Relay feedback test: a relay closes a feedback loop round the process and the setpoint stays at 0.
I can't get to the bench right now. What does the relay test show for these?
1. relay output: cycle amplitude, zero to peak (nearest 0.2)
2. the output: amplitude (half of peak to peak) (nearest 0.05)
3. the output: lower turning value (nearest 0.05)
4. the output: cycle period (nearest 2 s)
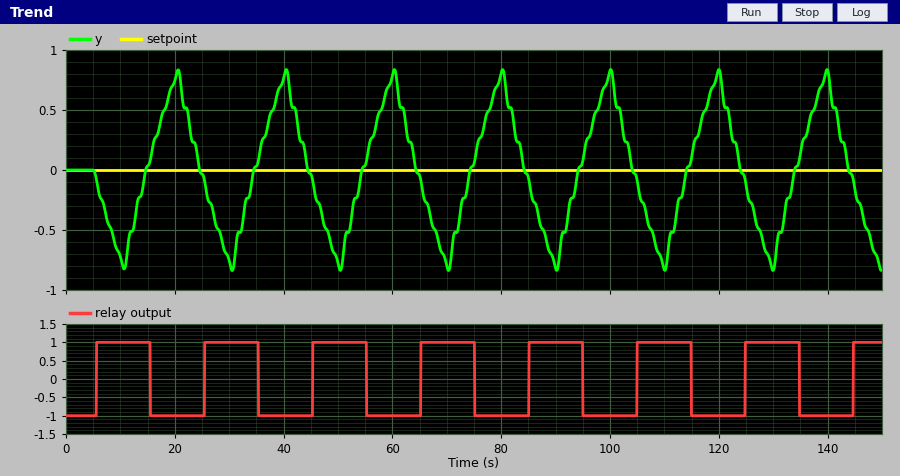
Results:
1.0
0.85
-0.85
20 s
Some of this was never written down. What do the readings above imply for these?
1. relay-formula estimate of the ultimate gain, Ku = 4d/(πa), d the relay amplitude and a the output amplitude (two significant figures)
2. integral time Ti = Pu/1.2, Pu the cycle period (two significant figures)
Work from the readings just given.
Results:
1.5
17 s
